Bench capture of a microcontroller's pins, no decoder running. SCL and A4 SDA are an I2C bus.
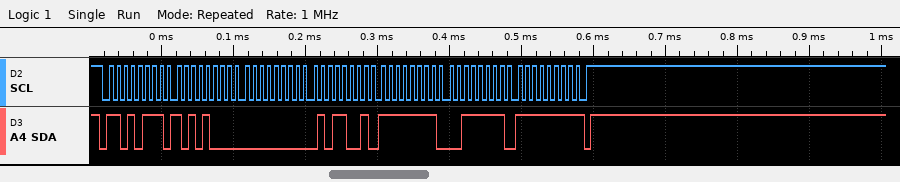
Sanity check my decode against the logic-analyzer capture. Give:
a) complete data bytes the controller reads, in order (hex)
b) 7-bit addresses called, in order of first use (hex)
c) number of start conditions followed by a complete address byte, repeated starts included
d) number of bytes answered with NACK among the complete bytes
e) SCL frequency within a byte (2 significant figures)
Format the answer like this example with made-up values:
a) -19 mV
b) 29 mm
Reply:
a) A8 00 59 FF 3F FF
b) 0x6B
c) 1
d) 1
e) 100 kHz
